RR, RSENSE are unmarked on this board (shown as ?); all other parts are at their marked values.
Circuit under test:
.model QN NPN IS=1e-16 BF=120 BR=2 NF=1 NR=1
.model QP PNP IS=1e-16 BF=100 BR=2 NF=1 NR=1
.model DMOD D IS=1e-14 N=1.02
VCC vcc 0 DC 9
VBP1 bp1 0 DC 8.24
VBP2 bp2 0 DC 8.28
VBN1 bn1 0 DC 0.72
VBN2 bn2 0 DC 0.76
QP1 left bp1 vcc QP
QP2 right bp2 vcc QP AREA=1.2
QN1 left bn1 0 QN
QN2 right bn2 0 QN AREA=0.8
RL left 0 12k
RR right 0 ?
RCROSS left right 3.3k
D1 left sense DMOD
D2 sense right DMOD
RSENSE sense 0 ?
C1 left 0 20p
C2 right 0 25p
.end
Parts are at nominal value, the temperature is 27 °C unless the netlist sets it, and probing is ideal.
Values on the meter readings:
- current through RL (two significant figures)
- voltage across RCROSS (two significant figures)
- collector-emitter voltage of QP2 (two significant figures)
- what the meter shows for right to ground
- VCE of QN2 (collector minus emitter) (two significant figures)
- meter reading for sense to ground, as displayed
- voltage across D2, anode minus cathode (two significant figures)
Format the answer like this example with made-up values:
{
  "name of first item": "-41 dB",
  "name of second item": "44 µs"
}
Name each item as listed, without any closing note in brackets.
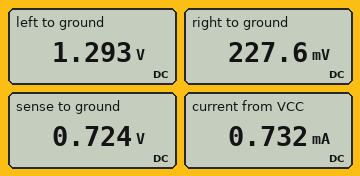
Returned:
{
  "current through RL": "110 µA",
  "voltage across RCROSS": "1.1 V",
  "collector-emitter voltage of QP2": "-8.8 V",
  "what the meter shows for right to ground": "227.6 mV",
  "VCE of QN2 (collector minus emitter)": "230 mV",
  "meter reading for sense to ground, as displayed": "0.724 V",
  "voltage across D2, anode minus cathode": "500 mV"
}
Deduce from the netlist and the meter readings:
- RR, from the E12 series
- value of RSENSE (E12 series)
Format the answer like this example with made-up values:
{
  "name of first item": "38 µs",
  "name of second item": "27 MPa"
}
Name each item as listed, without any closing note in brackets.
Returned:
{
  "RR, from the E12 series": "22 kΩ",
  "value of RSENSE": "33 kΩ"
}
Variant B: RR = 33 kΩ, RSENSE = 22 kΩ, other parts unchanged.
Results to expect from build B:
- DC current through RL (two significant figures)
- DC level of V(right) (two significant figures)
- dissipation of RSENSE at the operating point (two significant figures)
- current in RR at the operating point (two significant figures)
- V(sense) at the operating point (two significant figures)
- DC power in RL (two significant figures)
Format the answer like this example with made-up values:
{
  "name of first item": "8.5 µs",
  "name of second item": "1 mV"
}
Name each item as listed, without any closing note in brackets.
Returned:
{
  "DC current through RL": "100 µA",
  "DC level of V(right)": "190 mV",
  "dissipation of RSENSE at the operating point": "20 µW",
  "current in RR at the operating point": "5.9 µA",
  "V(sense) at the operating point": "670 mV",
  "DC power in RL": "130 µW"
}
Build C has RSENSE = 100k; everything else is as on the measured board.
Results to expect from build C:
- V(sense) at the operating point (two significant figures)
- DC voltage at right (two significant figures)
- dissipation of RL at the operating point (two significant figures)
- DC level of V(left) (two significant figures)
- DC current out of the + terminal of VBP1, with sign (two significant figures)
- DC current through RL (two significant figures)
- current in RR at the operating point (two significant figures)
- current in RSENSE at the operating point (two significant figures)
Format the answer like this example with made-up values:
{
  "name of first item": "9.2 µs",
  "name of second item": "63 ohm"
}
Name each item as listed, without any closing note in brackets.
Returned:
{
  "V(sense) at the operating point": "850 mV",
  "DC voltage at right": "330 mV",
  "dissipation of RL at the operating point": "160 µW",
  "DC level of V(left)": "1.4 V",
  "DC current out of the + terminal of VBP1, with sign": "-5.8 µA",
  "DC current through RL": "120 µA",
  "current in RR at the operating point": "15 µA",
  "current in RSENSE at the operating point": "8.5 µA"
}
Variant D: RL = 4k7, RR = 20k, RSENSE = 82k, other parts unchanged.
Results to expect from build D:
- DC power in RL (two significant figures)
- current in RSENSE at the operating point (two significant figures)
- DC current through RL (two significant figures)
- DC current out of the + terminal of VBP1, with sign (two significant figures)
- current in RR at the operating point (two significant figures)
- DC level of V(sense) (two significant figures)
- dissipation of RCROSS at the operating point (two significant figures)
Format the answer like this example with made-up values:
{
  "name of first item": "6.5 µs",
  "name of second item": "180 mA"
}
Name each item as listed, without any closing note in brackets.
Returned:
{
  "DC power in RL": "170 µW",
  "current in RSENSE at the operating point": "4.6 µA",
  "DC current through RL": "190 µA",
  "DC current out of the + terminal of VBP1, with sign": "-5.8 µA",
  "current in RR at the operating point": "2.9 µA",
  "DC level of V(sense)": "380 mV",
  "dissipation of RCROSS at the operating point": "220 µW"
}
